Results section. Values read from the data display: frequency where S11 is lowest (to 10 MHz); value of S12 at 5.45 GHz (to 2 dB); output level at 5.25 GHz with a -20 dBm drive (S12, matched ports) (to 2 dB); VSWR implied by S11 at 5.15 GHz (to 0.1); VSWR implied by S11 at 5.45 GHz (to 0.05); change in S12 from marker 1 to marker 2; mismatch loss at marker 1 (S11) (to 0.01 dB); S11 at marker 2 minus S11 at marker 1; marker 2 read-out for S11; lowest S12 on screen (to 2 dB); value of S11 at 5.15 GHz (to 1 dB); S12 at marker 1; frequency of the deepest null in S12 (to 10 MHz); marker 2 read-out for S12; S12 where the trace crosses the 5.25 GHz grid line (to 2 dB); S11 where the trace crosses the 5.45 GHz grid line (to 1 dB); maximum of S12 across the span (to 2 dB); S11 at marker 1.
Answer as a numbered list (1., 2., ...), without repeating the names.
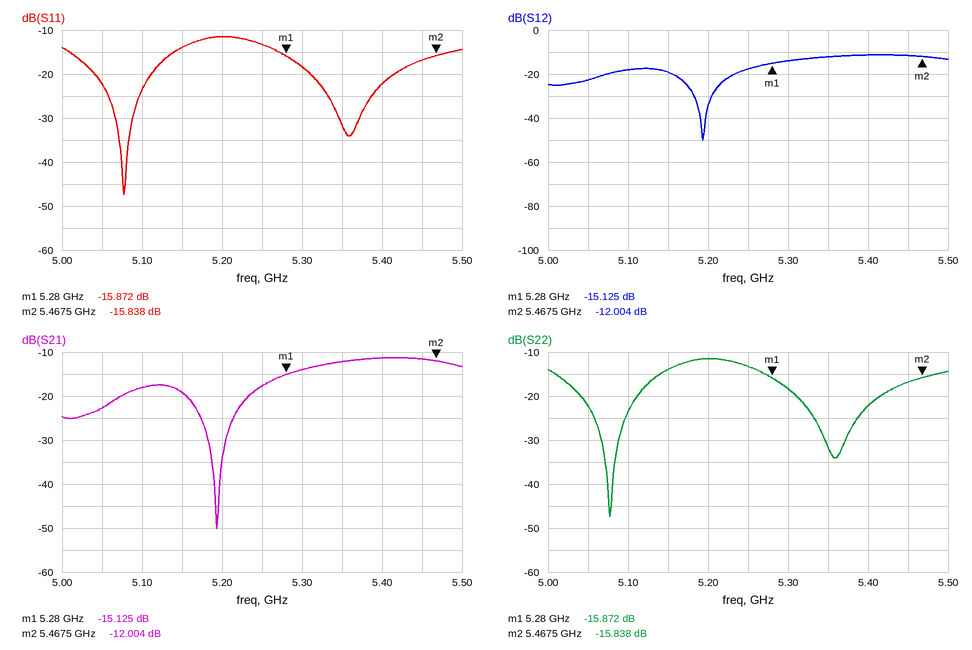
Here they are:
1. 5.08 GHz
2. -12 dB
3. -38 dBm
4. 1.5
5. 1.35
6. 3.121 dB
7. 0.11 dB
8. 0.034 dB
9. -15.838 dB
10. -50 dB
11. -14 dB
12. -15.125 dB
13. 5.19 GHz
14. -12.004 dB
15. -18 dB
16. -17 dB
17. -12 dB
18. -15.872 dB
